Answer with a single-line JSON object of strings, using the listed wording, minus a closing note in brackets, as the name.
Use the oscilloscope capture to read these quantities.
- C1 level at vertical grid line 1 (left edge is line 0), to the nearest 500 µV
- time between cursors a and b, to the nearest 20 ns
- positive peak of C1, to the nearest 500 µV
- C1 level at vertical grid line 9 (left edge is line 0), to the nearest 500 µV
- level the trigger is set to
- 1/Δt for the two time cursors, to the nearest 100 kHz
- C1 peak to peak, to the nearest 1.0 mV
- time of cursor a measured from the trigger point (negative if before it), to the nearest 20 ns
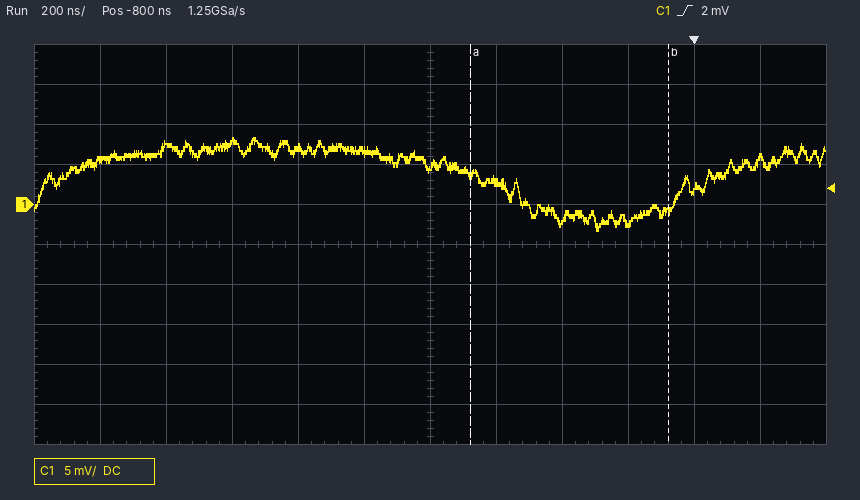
{"C1 level at vertical grid line 1 (left edge is line 0), to the nearest 500 µV": "5.5 mV", "time between cursors a and b, to the nearest 20 ns": "600 ns", "positive peak of C1, to the nearest 500 µV": "8.5 mV", "C1 level at vertical grid line 9 (left edge is line 0), to the nearest 500 µV": "-2.5 mV", "level the trigger is set to": "2 mV", "1/Δt for the two time cursors, to the nearest 100 kHz": "1.7 MHz", "C1 peak to peak, to the nearest 1.0 mV": "12.0 mV", "time of cursor a measured from the trigger point (negative if before it), to the nearest 20 ns": "-680 ns"}
